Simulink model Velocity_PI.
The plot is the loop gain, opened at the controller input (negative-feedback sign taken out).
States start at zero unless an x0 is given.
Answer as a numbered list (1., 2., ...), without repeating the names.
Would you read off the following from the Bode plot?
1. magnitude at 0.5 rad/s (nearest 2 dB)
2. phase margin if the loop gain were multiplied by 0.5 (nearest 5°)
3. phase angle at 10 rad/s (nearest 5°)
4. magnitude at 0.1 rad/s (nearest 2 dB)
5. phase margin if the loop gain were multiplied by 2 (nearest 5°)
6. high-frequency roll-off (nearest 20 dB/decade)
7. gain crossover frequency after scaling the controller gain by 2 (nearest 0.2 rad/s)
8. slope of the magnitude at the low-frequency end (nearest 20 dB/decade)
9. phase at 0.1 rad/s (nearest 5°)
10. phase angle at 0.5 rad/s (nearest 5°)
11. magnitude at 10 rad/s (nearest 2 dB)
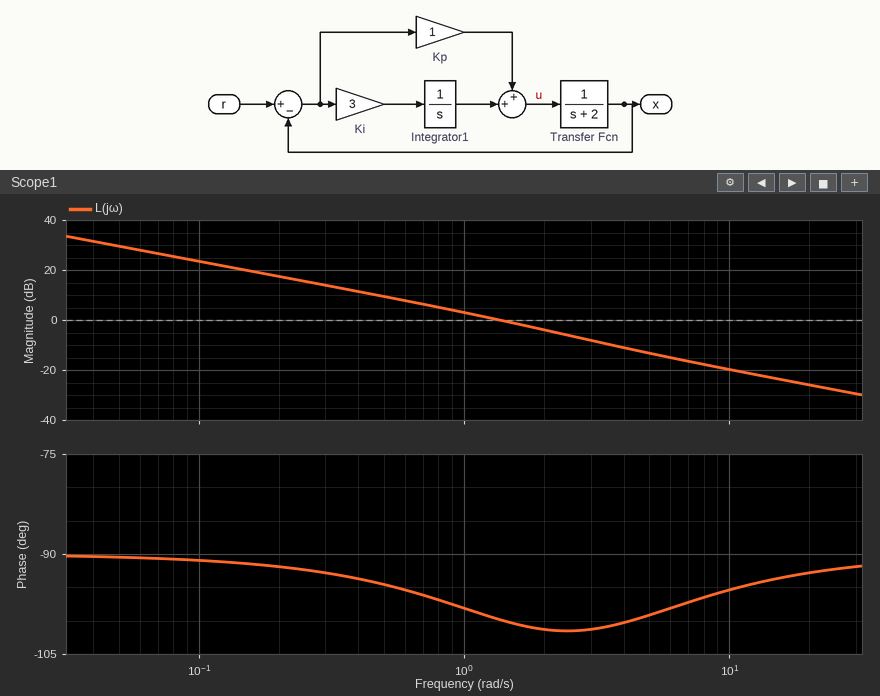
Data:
1. 10 dB
2. 85°
3. -95°
4. 24 dB
5. 80°
6. -20 dB/decade
7. 2.4 rad/s
8. -20 dB/decade
9. -90°
10. -95°
11. -20 dB
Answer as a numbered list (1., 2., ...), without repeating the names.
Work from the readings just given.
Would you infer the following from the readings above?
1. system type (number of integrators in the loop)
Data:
1. 1
